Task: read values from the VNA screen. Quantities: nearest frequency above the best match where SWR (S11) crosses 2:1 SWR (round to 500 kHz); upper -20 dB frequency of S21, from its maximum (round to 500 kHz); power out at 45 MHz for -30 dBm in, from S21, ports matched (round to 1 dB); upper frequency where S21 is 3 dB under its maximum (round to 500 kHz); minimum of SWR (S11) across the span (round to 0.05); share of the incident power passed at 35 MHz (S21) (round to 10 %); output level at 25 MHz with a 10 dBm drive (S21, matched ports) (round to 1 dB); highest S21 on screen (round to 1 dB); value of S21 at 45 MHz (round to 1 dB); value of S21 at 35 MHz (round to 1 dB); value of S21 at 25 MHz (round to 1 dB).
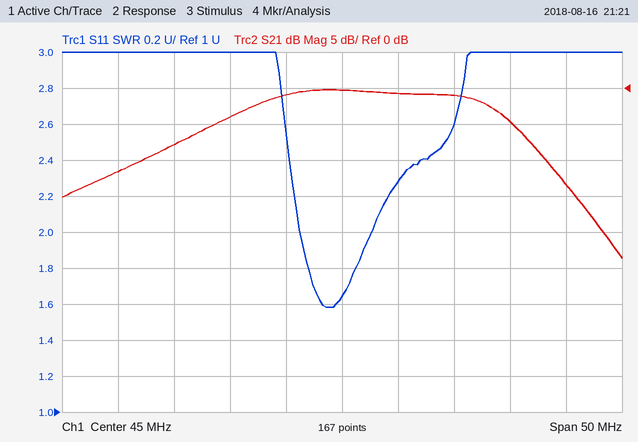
47.5 MHz
68.5 MHz
-30 dBm
59.0 MHz
1.60
40 %
-2 dBm
0 dB
0 dB
-4 dB
-12 dB
